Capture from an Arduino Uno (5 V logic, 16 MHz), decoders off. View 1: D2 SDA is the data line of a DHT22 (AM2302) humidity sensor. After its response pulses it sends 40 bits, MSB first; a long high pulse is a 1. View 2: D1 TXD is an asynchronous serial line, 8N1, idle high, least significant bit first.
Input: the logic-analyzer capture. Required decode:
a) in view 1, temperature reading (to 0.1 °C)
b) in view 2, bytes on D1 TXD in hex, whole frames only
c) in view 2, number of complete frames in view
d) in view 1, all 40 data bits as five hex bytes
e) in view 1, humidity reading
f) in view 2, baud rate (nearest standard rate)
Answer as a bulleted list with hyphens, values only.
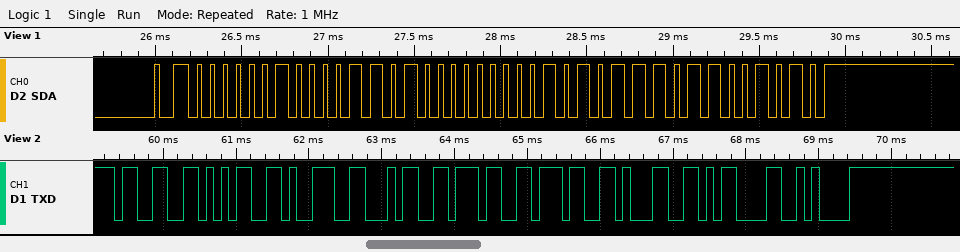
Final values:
- 17.4 °C
- 33 35 39 34 37 37 31 0D 0A
- 9
- 02 1A 00 AE CA
- 53.8 %
- 9600 baud
